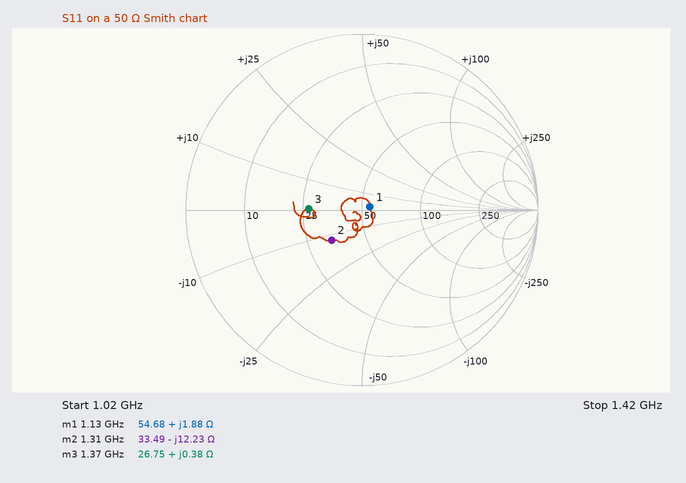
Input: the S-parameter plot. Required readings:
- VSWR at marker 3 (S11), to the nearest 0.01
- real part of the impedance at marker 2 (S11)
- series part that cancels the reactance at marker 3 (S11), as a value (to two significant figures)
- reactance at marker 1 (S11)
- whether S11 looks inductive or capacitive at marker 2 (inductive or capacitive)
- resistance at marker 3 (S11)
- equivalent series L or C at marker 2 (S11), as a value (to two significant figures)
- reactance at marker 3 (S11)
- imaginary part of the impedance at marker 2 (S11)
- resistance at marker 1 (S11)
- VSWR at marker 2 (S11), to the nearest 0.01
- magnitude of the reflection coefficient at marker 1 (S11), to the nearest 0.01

1.87
33.49 Ω
310 pF
+1.88 Ω
capacitive
26.75 Ω
9.9 pF
+0.38 Ω
-12.23 Ω
54.68 Ω
1.64
0.05
